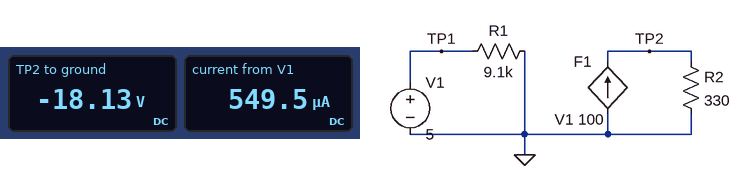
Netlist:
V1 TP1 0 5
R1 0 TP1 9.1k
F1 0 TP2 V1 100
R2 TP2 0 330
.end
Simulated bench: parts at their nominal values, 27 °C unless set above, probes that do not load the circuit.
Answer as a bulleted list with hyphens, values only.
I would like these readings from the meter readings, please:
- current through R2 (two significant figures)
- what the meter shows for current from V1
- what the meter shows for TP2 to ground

- 55 mA
- 549.5 µA
- -18.13 V
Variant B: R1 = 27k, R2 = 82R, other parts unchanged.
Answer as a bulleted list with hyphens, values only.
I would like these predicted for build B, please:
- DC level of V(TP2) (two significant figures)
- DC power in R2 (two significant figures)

- -1.5 V
- 28 mW
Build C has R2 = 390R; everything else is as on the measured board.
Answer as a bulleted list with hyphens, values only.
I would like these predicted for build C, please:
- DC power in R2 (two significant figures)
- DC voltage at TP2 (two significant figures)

- 1.2 W
- -21 V
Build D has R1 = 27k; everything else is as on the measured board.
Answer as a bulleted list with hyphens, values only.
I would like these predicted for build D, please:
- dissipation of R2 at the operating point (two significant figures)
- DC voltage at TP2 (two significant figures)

- 110 mW
- -6.1 V
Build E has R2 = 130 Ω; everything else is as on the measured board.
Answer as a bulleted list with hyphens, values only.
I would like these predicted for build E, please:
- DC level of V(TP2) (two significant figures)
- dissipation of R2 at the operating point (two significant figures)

- -7.1 V
- 390 mW
